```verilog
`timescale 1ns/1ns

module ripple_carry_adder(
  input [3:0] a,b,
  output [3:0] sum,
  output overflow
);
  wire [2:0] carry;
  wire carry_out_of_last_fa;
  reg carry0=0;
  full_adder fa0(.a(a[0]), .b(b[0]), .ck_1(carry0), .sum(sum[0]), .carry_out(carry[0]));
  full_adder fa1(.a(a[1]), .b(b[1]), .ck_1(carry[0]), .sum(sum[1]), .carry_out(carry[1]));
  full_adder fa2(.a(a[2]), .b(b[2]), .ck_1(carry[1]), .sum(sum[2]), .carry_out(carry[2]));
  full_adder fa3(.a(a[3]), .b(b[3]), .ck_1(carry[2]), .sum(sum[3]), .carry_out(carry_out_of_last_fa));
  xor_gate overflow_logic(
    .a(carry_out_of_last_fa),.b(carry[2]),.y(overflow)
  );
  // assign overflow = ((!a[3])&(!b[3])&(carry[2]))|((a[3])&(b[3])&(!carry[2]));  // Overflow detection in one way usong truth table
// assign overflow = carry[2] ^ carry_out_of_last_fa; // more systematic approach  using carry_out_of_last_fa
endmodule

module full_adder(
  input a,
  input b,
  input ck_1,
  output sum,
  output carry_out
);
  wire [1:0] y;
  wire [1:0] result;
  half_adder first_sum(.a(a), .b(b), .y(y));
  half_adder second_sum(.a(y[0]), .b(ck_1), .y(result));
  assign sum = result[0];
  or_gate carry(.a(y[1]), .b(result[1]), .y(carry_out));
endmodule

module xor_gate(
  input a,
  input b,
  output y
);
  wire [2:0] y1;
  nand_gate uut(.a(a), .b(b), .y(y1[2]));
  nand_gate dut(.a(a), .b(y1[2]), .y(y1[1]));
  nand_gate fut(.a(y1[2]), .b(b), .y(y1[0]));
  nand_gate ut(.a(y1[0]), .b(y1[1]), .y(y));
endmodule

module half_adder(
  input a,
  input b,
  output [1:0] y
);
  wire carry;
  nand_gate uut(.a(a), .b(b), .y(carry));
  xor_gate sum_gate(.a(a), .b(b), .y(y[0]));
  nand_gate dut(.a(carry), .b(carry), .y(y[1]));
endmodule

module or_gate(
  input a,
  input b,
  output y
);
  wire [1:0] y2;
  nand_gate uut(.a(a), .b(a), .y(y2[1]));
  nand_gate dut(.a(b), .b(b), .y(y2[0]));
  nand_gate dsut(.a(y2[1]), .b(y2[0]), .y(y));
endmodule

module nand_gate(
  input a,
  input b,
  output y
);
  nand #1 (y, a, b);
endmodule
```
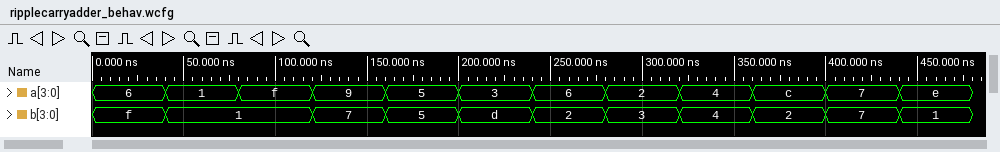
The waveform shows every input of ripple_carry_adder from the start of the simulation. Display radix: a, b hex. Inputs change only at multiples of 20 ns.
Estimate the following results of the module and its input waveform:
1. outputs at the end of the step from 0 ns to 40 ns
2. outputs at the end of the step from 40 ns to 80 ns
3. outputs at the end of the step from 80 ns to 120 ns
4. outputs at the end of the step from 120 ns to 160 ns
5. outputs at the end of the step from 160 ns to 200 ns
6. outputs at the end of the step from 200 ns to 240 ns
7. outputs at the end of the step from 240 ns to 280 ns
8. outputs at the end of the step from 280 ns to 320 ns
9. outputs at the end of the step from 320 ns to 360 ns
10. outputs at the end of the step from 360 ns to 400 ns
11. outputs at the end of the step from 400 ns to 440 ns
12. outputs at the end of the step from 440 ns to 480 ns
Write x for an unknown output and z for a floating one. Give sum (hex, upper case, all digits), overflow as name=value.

sum=5, overflow=0
sum=2, overflow=0
sum=0, overflow=0
sum=0, overflow=0
sum=A, overflow=1
sum=0, overflow=0
sum=8, overflow=1
sum=5, overflow=0
sum=8, overflow=1
sum=E, overflow=0
sum=E, overflow=1
sum=F, overflow=0
